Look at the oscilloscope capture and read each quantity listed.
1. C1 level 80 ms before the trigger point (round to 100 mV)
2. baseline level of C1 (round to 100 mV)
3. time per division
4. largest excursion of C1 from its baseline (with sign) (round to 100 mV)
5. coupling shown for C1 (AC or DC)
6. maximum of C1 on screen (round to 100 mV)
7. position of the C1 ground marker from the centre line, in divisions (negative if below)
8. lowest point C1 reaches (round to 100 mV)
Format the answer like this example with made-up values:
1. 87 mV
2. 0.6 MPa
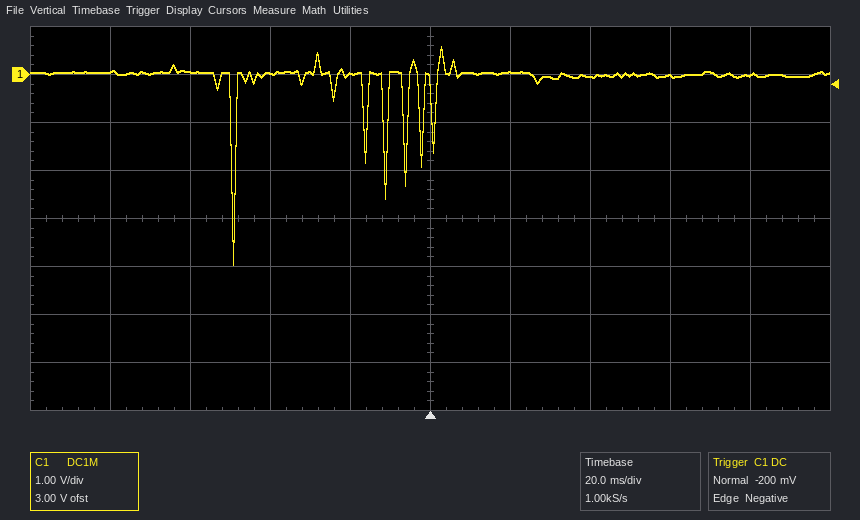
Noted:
1. 100 mV
2. 0.0 V
3. 20 ms
4. -4.0 V
5. DC
6. 600 mV
7. +3.0 div
8. -4.0 V
